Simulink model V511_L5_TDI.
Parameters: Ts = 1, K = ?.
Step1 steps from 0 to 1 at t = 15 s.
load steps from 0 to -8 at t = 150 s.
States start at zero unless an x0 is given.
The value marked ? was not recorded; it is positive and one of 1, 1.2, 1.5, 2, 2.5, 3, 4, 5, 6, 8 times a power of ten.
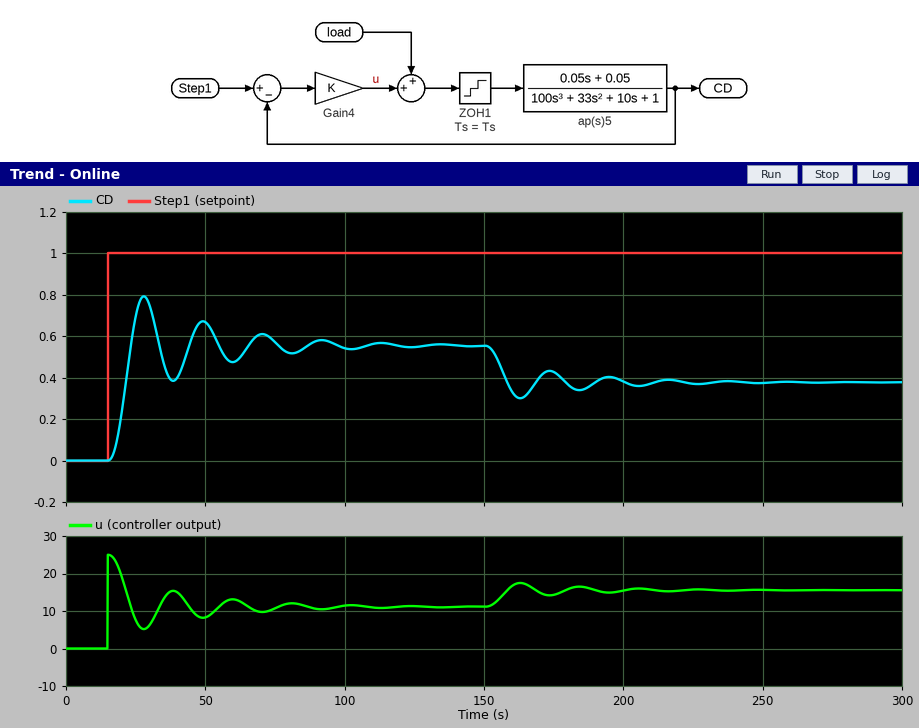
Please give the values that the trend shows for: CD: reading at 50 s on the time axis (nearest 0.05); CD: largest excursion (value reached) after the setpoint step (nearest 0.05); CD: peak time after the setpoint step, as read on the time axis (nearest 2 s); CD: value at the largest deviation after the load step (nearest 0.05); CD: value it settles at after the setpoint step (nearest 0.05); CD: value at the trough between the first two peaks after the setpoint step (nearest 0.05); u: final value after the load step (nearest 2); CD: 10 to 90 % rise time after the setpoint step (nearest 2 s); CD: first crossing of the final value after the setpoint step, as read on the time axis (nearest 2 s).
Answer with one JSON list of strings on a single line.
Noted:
["0.65", "0.80", "28 s", "0.30", "0.55", "0.40", "16", "6 s", "24 s"]
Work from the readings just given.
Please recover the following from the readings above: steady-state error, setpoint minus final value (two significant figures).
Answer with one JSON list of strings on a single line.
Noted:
["0.45"]
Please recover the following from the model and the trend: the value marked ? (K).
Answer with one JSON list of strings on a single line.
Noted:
["25"]
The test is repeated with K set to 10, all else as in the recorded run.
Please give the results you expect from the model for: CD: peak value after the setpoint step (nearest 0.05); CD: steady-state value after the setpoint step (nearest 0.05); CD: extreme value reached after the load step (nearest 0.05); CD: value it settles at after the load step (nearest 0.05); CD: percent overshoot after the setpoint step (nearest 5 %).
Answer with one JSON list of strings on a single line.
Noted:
["0.40", "0.35", "0.00", "0.05", "20 %"]
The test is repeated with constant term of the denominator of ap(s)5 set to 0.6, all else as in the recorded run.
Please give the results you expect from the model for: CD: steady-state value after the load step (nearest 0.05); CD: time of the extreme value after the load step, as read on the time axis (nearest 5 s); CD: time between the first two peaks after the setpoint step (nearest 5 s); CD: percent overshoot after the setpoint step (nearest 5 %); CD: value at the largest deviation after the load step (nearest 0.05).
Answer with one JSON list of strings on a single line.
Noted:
["0.45", "165 s", "20 s", "30 %", "0.40"]
